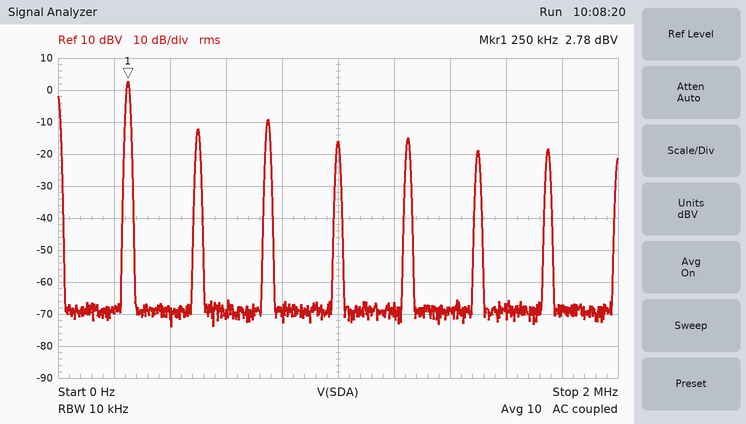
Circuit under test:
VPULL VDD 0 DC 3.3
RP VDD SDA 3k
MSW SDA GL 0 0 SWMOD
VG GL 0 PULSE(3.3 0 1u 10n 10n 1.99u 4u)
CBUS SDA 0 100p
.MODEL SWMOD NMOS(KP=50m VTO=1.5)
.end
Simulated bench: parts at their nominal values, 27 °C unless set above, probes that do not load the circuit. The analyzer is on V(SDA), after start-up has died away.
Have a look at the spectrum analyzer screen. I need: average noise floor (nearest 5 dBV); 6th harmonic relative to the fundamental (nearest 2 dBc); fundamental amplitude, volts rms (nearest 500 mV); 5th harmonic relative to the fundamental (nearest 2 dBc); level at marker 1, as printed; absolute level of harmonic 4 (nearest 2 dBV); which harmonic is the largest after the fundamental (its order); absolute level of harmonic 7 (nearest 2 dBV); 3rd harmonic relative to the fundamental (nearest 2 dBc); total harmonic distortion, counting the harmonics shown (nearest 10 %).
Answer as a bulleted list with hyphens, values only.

- -70 dBV
- -22 dBc
- 1.5 V
- -18 dBc
- 2.78 dBV
- -16 dBV
- 3
- -18 dBV
- -12 dBc
- 40 %
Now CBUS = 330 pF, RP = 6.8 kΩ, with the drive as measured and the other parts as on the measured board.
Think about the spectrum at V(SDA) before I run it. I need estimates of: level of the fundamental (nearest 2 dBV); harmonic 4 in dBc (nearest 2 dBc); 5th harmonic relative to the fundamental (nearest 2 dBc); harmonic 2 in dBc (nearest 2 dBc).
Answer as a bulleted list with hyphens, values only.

- -4 dBV
- -14 dBc
- -16 dBc
- -8 dBc
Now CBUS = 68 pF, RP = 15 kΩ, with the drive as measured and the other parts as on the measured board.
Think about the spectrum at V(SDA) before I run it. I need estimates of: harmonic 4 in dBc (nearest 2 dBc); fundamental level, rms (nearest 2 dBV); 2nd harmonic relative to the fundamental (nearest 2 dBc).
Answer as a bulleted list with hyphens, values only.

- -16 dBc
- 0 dBV
- -10 dBc
